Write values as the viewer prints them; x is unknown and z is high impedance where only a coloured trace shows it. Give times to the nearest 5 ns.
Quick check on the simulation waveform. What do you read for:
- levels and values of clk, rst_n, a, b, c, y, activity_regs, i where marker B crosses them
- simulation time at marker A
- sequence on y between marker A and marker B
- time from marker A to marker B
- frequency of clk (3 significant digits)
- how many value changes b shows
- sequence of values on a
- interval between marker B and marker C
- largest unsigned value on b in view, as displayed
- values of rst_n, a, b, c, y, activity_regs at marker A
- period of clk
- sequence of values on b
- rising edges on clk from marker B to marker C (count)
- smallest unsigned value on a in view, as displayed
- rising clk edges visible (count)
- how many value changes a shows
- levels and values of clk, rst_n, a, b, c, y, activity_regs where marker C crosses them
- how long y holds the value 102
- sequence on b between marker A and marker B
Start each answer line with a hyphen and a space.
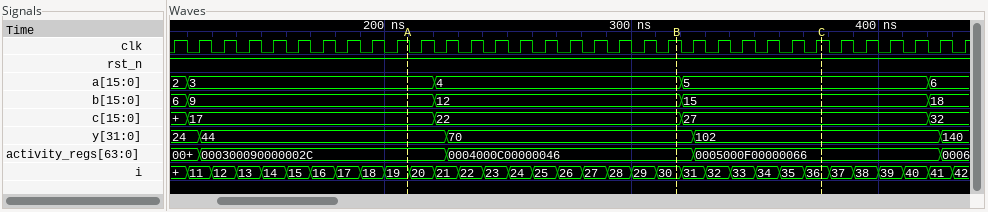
- clk=1, rst_n=1, a=4, b=12, c=22, y=70, activity_regs=0004000C00000046, i=30
- 210 ns
- 44, 70
- 110 ns
- 100 MHz
- 4
- 2, 3, 4, 5, 6
- 60 ns
- 18
- rst_n=1, a=3, b=9, c=17, y=44, activity_regs=000300090000002C
- 10 ns
- 6, 9, 12, 15, 18
- 6
- 2
- 33
- 4
- clk=1, rst_n=1, a=5, b=15, c=27, y=102, activity_regs=0005000F00000066
- 100 ns
- 9, 12
